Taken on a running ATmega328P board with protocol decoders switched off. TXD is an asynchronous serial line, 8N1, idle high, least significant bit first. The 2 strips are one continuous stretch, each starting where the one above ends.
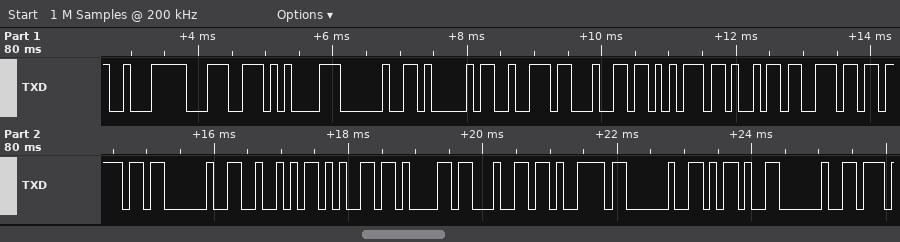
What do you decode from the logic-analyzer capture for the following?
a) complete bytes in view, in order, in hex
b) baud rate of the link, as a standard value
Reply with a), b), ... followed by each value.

a) 0xE2 0x9C 0x85 0x20 0x41 0x72 0x64 0x75 0x69 0x6E 0x6F 0x20 0x52 0x65 0x61 0x64 0x79 0x20 0x2D 0x20
b) 9600 baud
